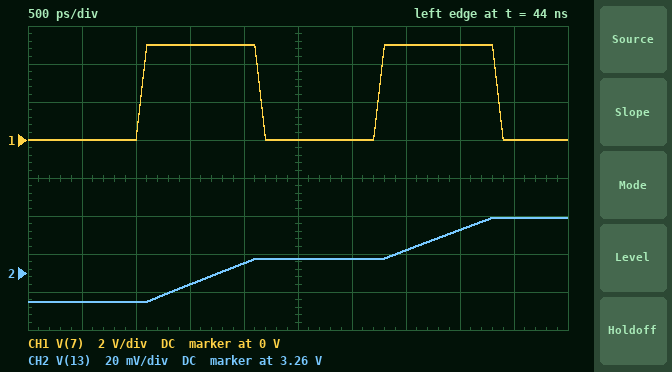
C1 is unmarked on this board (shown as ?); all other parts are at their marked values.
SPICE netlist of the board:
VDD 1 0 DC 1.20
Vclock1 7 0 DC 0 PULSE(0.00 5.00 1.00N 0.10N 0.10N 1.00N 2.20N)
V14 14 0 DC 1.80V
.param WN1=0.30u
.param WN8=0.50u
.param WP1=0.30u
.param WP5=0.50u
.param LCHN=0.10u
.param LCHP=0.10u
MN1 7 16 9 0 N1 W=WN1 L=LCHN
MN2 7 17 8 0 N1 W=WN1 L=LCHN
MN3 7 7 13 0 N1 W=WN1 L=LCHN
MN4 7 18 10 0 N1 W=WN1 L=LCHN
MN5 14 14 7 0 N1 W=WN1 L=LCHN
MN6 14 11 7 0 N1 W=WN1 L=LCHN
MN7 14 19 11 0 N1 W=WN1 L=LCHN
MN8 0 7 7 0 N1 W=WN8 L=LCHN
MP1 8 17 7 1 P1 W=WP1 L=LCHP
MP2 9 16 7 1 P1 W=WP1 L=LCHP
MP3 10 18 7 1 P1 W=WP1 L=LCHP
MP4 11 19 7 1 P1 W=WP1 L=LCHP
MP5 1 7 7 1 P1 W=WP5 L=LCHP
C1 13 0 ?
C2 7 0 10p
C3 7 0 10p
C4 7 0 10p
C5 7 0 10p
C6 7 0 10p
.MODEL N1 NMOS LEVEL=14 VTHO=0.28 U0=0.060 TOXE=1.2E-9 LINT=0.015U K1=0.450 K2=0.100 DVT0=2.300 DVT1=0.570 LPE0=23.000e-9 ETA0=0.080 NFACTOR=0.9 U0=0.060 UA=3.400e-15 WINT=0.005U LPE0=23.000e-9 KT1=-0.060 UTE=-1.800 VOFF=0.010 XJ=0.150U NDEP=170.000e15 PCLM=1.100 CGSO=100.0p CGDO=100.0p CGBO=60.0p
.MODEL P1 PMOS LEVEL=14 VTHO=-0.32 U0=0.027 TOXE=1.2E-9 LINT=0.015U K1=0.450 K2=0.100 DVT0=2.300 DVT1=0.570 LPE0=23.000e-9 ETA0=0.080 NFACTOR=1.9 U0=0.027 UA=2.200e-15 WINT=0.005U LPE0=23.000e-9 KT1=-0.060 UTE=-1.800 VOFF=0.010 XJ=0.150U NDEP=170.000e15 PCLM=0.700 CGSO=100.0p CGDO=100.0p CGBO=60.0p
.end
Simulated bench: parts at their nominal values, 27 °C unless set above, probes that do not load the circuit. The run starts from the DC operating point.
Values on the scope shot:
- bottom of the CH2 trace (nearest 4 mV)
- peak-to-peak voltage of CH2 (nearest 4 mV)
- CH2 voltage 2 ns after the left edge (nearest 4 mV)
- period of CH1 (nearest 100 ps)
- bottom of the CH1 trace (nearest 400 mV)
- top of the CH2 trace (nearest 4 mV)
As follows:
3.244 V
44 mV
3.264 V
2.2 ns
0 V
3.288 V
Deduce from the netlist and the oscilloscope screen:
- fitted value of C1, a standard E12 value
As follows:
22 pF
